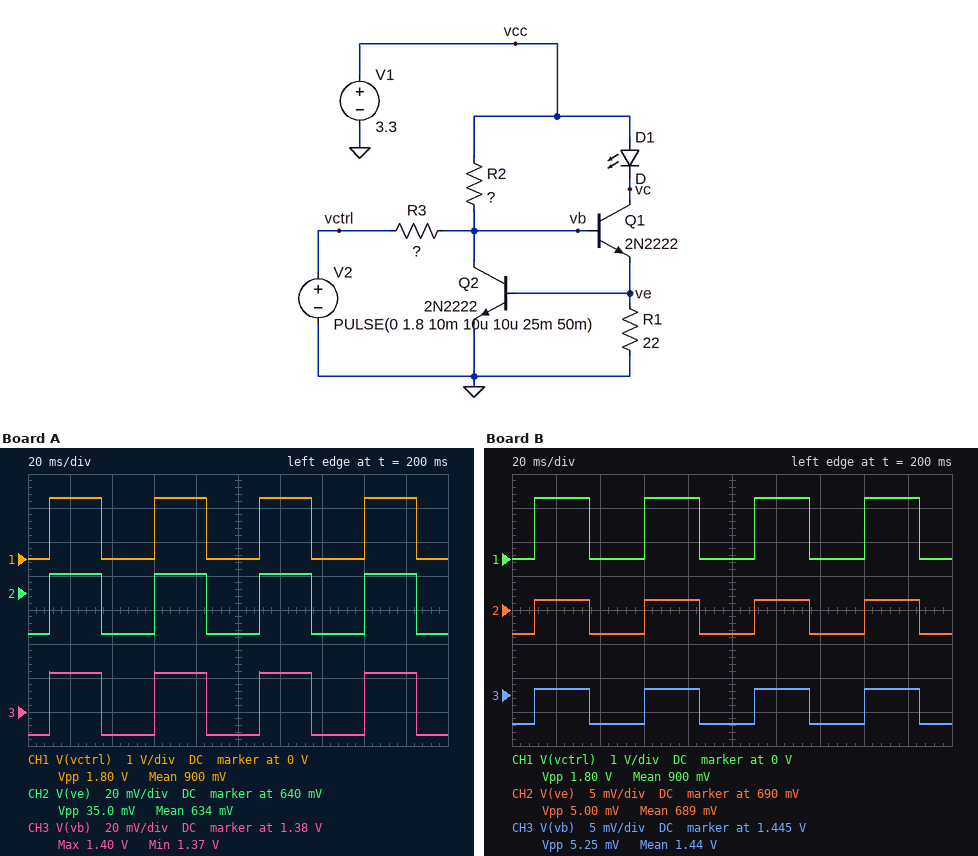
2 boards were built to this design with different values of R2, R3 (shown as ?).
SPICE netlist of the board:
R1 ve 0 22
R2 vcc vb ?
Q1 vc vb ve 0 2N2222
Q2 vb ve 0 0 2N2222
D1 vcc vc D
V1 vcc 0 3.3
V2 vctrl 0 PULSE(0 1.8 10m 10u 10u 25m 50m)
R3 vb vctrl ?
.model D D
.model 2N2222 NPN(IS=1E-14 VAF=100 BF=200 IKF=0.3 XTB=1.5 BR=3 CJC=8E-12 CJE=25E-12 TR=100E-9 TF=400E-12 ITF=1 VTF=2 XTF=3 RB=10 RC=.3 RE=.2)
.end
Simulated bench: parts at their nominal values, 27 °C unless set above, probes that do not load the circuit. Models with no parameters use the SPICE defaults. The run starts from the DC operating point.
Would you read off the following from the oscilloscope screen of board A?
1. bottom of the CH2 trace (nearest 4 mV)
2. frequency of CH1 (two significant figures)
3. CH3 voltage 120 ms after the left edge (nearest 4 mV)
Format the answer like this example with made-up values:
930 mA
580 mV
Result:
616 mV
20 Hz
1.404 V
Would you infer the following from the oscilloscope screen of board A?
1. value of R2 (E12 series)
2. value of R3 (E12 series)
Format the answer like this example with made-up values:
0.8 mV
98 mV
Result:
2.2 kΩ
2.7 kΩ
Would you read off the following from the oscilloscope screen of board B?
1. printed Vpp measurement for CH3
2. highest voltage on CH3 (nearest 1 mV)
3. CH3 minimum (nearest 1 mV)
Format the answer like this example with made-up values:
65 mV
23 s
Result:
5.25 mV
1.446 V
1.441 V
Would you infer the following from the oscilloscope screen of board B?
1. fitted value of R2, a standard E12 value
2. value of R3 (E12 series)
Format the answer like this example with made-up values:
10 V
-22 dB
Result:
470 Ω
2.7 kΩ
